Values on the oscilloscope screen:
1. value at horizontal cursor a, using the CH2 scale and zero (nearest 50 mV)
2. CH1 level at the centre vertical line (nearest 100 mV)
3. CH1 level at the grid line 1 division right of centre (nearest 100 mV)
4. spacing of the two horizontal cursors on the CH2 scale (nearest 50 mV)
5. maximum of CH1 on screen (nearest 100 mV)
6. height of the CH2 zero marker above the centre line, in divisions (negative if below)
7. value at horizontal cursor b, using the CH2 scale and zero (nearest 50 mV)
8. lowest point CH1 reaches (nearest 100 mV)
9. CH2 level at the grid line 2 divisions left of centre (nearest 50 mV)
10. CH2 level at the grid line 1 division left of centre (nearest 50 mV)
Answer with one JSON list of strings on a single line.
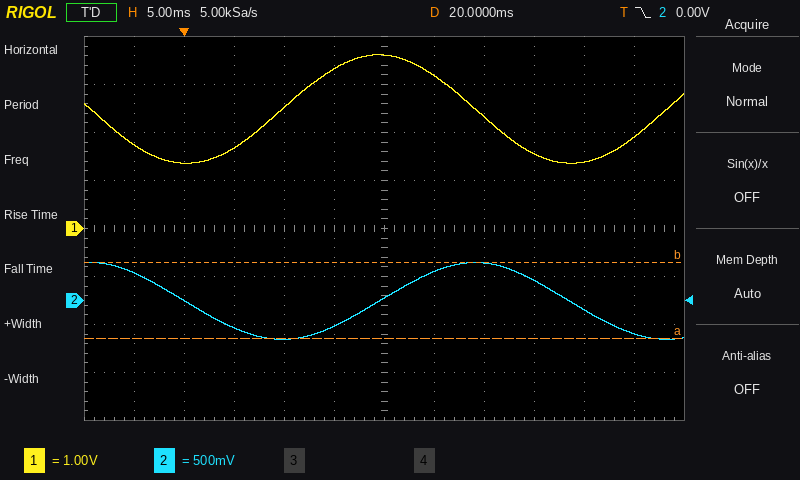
["-400 mV", "3.6 V", "3.2 V", "800 mV", "3.6 V", "-1.5 div", "400 mV", "1.4 V", "-400 mV", "-250 mV"]
